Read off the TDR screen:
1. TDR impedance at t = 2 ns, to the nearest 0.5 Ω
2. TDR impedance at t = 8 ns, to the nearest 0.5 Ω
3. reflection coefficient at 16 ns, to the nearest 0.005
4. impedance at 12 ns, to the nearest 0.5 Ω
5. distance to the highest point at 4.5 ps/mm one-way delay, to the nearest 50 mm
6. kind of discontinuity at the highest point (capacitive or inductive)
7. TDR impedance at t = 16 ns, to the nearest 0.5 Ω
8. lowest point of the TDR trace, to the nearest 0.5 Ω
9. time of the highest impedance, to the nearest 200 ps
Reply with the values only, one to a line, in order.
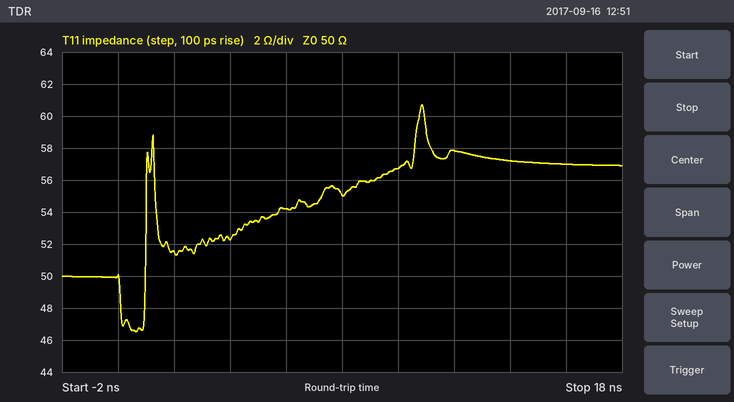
51.5 Ω
55.0 Ω
+0.065
58.0 Ω
1.20 m
inductive
57.0 Ω
46.5 Ω
10.8 ns
